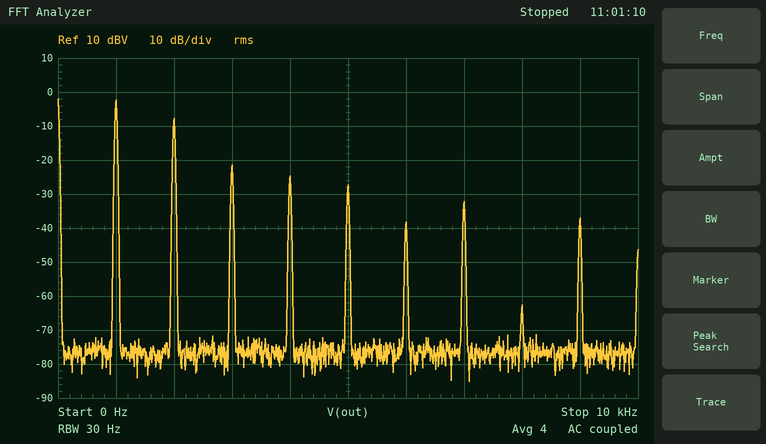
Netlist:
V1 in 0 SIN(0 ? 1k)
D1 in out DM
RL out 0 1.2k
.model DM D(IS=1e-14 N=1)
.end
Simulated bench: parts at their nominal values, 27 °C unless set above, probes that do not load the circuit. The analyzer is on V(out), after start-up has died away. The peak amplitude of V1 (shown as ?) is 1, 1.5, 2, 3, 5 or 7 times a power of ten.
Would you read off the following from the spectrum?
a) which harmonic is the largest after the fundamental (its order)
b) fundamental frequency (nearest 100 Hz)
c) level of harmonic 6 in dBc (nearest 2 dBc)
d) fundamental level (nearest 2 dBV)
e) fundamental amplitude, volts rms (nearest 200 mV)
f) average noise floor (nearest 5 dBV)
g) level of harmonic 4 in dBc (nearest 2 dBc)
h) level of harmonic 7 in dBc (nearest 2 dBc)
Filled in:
2
1.0 kHz
-36 dBc
-2 dBV
800 mV
-75 dBV
-22 dBc
-30 dBc
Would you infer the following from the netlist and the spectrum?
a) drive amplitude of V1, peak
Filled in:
3 V
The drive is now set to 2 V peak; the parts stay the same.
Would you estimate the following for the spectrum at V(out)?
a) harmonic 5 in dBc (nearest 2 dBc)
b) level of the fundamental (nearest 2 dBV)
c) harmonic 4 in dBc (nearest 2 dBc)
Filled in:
-22 dBc
-8 dBV
-26 dBc
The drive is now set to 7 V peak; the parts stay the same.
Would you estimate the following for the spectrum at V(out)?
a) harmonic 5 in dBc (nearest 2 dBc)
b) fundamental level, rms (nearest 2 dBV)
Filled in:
-32 dBc
6 dBV
